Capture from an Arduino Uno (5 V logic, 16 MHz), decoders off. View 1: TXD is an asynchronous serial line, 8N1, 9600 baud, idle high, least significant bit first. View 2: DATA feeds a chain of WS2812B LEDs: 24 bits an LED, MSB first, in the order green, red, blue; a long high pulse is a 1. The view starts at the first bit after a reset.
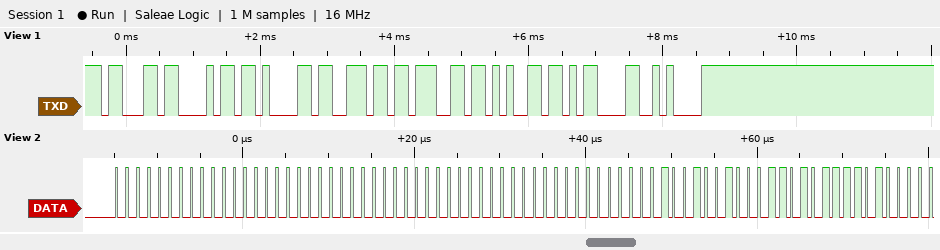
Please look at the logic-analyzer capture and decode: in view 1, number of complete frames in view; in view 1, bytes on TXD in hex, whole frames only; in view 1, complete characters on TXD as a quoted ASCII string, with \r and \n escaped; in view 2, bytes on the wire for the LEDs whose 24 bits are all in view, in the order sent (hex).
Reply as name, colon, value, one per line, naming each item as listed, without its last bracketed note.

in view 1, number of complete frames in view: 8
in view 1, bytes on TXD in hex, whole frames only: 0x63 0x68 0x61 0x6E 0x67 0x65 0x0D 0x0A
in view 1, complete characters on TXD as a quoted ASCII string, with \r and \n escaped: "change\r\n"
in view 2, bytes on the wire for the LEDs whose 24 bits are all in view, in the order sent: 00 00 00 00 00 00 12 46 BD
